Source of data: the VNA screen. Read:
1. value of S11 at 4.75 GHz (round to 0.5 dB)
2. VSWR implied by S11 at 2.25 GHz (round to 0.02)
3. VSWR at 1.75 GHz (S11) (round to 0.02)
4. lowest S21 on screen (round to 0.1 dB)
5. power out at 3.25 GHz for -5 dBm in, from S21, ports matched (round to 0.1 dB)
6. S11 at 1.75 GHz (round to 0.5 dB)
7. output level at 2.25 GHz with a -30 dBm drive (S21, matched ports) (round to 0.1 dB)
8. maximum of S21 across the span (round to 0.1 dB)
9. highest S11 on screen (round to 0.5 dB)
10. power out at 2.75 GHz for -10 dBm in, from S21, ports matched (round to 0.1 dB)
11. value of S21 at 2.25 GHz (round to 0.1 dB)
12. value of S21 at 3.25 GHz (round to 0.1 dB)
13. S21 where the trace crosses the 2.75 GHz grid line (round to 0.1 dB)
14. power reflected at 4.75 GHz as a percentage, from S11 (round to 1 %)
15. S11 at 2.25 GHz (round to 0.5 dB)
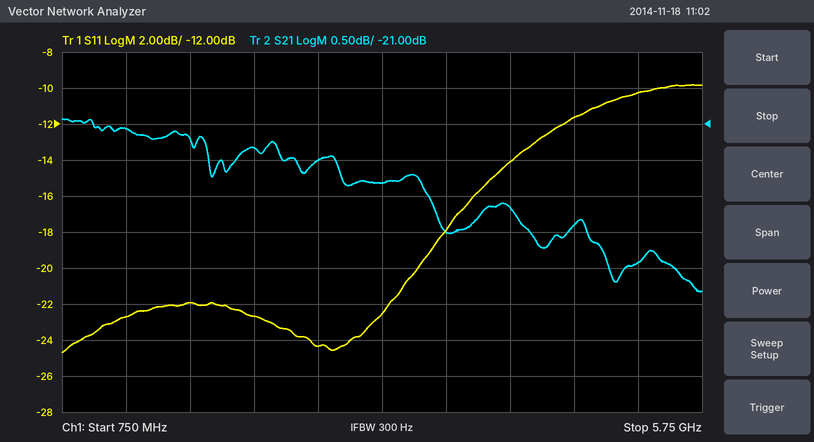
-11.5 dB
1.16
1.18
-23.3 dB
-26.8 dBm
-22.0 dB
-51.3 dBm
-20.9 dB
-10.0 dB
-31.5 dBm
-21.3 dB
-21.8 dB
-21.5 dB
7 %
-22.5 dB
